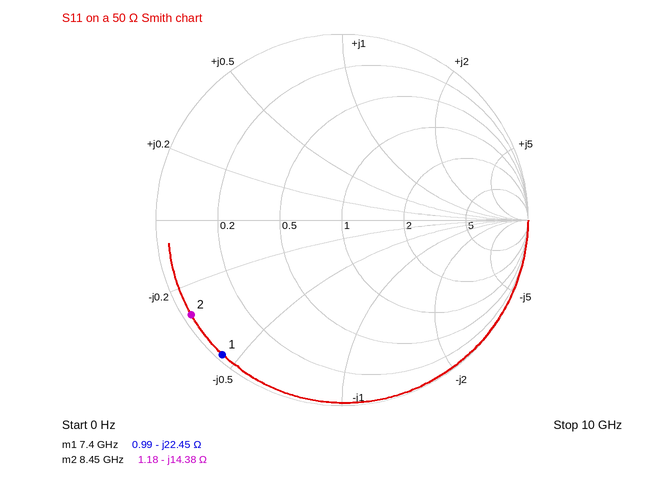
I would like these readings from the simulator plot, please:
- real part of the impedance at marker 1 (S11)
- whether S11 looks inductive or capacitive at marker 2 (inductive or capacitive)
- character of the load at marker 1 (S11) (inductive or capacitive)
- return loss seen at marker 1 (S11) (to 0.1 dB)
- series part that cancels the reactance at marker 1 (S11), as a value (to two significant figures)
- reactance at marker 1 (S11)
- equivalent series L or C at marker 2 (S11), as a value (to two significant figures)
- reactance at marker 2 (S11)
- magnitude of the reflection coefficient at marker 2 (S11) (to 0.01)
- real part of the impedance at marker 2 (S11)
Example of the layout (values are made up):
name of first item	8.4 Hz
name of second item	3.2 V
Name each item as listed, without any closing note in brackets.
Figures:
real part of the impedance at marker 1	0.99 Ω
whether S11 looks inductive or capacitive at marker 2	capacitive
character of the load at marker 1 (S11)	capacitive
return loss seen at marker 1 (S11)	0.3 dB
series part that cancels the reactance at marker 1 (S11), as a value	480 pH
reactance at marker 1	-22.45 Ω
equivalent series L or C at marker 2 (S11), as a value	1.3 pF
reactance at marker 2	-14.38 Ω
magnitude of the reflection coefficient at marker 2 (S11)	0.96
real part of the impedance at marker 2	1.18 Ω
